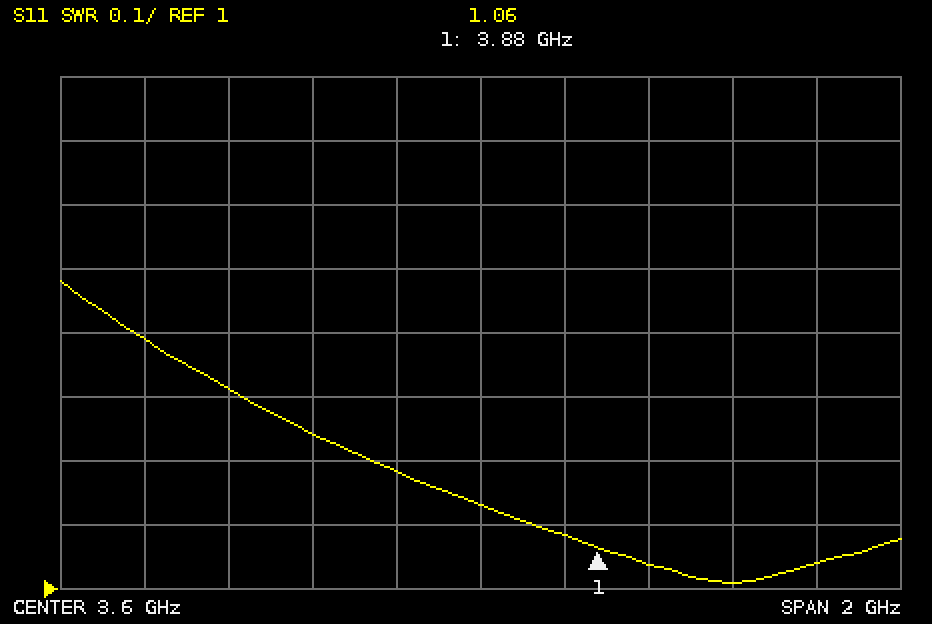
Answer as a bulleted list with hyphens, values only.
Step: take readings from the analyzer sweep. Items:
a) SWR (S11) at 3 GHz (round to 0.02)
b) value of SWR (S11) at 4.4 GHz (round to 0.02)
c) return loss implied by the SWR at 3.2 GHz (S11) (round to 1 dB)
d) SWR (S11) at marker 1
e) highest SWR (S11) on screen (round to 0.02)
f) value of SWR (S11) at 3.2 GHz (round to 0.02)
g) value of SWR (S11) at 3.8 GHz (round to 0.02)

- 1.32
- 1.04
- 19 dB
- 1.06
- 1.48
- 1.24
- 1.08
